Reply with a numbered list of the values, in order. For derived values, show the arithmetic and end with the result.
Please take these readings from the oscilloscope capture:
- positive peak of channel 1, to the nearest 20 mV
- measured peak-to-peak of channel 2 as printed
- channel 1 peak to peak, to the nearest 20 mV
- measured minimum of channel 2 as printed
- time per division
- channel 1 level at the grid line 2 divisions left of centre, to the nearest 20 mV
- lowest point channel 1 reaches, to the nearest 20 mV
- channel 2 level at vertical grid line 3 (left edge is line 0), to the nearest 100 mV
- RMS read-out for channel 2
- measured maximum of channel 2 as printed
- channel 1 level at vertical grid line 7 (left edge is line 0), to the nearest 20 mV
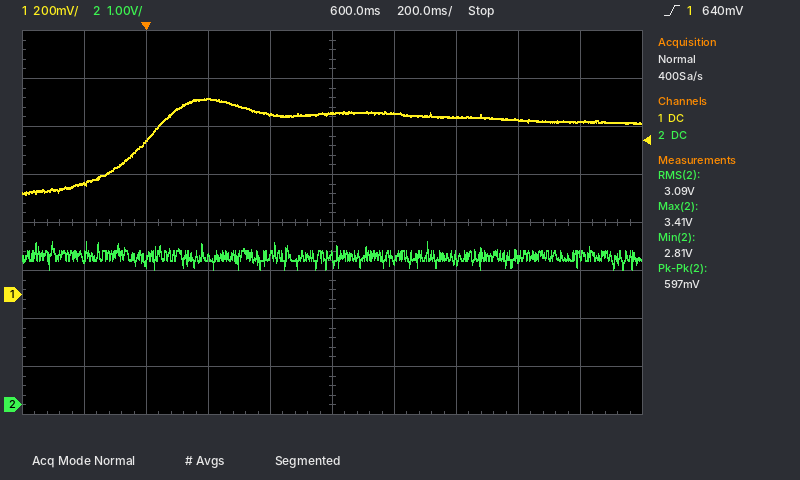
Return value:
1. 820 mV
2. 597 mV
3. 820 mV − (420 mV) = 400 mV
4. 2.81 V
5. 200 ms
6. 820 mV
7. 420 mV
8. 3.1 V
9. 3.09 V
10. 3.41 V
11. 740 mV
